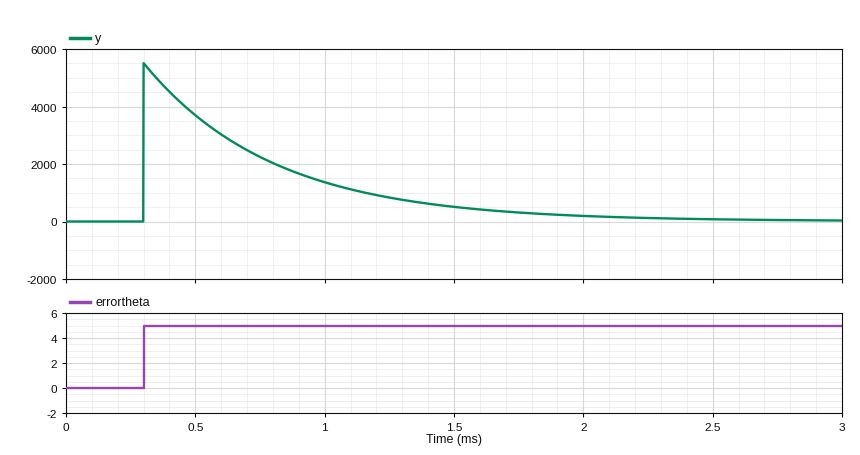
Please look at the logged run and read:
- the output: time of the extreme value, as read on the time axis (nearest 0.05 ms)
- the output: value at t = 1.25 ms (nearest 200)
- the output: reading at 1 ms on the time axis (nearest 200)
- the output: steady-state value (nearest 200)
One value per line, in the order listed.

0.30 ms
800
1400
0
